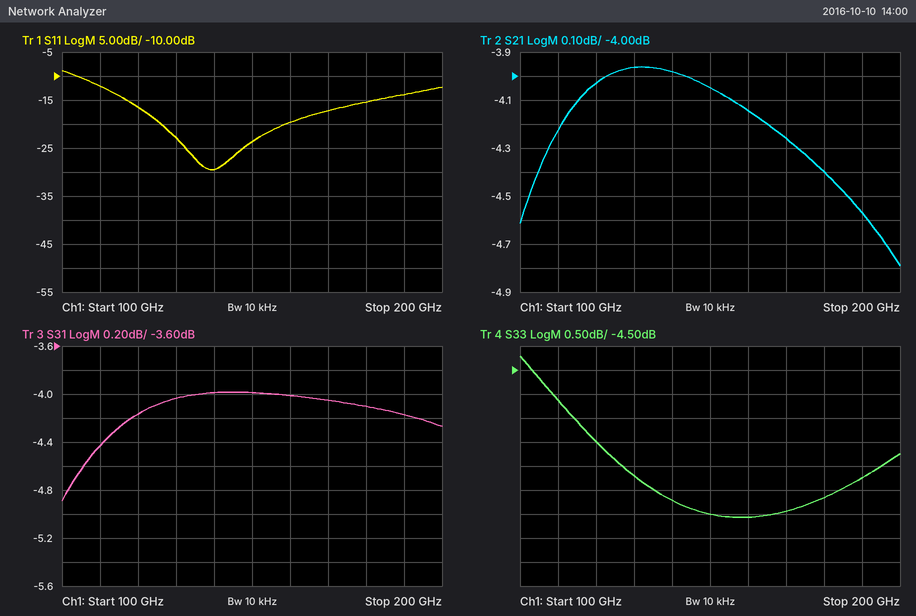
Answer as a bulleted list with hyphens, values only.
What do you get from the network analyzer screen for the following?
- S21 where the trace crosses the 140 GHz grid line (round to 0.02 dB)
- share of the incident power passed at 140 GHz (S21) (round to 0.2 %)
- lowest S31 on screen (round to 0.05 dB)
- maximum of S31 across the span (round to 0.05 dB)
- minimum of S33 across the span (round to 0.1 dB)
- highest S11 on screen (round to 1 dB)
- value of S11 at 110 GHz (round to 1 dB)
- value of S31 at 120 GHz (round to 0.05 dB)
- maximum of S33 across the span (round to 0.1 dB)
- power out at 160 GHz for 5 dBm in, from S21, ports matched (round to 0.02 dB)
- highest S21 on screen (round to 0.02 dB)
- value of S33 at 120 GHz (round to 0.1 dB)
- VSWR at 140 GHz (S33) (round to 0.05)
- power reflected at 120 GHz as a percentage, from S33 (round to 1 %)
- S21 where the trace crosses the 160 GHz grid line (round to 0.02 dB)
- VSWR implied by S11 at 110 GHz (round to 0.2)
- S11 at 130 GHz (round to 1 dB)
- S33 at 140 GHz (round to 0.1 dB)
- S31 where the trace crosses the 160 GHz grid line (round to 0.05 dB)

- -3.98 dB
- 40.0 %
- -4.90 dB
- -4.00 dB
- -7.6 dB
- -9 dB
- -12 dB
- -4.15 dB
- -4.2 dB
- 0.86 dBm
- -3.96 dB
- -6.0 dB
- 2.55
- 25 %
- -4.14 dB
- 1.6
- -23 dB
- -7.2 dB
- -4.00 dB
